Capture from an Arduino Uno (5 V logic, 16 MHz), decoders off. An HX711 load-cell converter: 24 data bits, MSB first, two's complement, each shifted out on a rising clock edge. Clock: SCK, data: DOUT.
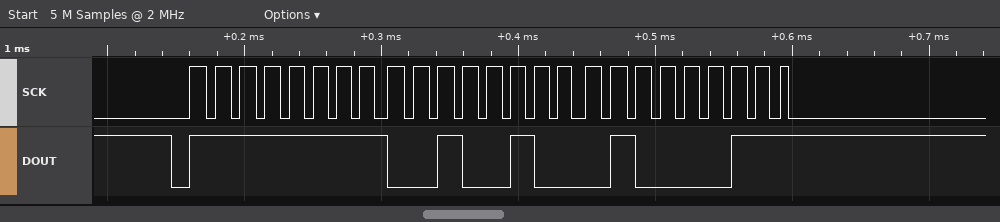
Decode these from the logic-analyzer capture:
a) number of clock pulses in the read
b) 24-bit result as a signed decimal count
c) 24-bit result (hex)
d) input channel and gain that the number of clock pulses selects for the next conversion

25
-56253
0xFF2443
channel A, gain 128
